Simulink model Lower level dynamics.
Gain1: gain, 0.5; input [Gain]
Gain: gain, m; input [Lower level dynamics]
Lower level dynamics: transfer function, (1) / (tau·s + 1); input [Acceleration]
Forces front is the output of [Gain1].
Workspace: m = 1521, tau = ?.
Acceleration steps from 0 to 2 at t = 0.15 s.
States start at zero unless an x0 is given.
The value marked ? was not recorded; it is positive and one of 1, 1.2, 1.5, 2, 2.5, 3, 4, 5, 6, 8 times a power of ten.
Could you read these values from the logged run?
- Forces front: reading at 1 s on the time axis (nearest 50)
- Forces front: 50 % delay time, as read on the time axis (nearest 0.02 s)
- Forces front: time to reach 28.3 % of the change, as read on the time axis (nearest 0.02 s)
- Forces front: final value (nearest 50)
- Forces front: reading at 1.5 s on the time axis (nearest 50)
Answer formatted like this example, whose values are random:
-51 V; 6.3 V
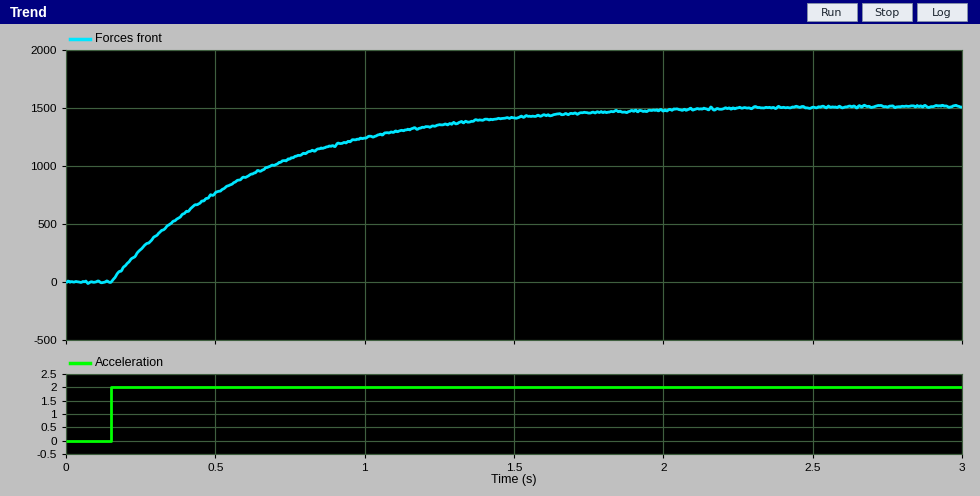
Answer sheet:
1250; 0.50 s; 0.32 s; 1500; 1400
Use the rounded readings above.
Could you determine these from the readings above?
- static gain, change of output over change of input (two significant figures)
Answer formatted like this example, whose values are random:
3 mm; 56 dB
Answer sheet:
750
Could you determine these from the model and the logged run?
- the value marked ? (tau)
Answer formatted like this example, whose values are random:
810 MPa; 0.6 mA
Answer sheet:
0.5
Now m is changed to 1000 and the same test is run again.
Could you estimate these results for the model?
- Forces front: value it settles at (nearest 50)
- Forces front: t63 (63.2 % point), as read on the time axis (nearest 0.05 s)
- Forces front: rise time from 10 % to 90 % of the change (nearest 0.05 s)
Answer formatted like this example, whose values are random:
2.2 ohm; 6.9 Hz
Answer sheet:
1000; 0.65 s; 1.10 s
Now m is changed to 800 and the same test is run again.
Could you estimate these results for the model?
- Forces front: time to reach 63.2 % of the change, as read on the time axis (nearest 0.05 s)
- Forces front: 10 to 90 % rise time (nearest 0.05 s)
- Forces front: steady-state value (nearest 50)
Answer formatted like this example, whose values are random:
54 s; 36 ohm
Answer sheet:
0.65 s; 1.10 s; 800
